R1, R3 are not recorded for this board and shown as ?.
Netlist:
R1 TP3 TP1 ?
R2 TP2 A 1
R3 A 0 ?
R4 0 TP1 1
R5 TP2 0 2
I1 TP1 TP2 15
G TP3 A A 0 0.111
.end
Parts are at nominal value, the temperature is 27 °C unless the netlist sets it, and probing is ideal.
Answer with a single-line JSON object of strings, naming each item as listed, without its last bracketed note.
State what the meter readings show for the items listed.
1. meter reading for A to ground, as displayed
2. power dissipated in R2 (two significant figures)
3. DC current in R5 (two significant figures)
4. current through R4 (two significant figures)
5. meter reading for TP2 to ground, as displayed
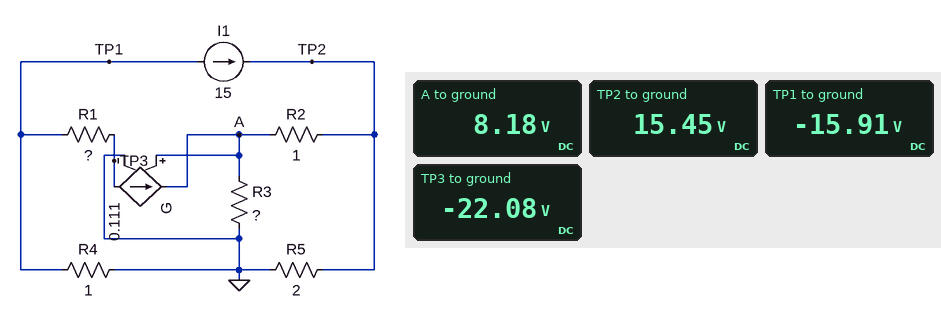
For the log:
{"meter reading for A to ground, as displayed": "8.18 V", "power dissipated in R2": "53 W", "DC current in R5": "7.7 A", "current through R4": "16 A", "meter reading for TP2 to ground, as displayed": "15.45 V"}
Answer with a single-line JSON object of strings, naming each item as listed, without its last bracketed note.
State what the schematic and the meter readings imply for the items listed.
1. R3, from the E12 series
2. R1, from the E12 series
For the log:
{"R3, from the E12 series": "1 Ω", "R1, from the E12 series": "6.8 Ω"}
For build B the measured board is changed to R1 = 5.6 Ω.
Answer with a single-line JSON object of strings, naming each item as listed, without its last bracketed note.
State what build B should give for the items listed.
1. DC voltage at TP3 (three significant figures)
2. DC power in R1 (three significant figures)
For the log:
{"DC voltage at TP3": "-21.0 V", "DC power in R1": "4.62 W"}
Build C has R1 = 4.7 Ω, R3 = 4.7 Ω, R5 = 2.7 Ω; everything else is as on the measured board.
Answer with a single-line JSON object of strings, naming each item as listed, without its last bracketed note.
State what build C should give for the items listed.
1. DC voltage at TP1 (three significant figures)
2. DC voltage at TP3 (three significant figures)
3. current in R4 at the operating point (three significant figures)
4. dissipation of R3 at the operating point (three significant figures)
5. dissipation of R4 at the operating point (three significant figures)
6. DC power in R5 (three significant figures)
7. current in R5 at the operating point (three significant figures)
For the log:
{"DC voltage at TP1": "-18.3 V", "DC voltage at TP3": "-33.6 V", "current in R4 at the operating point": "18.3 A", "dissipation of R3 at the operating point": "184 W", "dissipation of R4 at the operating point": "334 W", "DC power in R5": "389 W", "current in R5 at the operating point": "12.0 A"}
